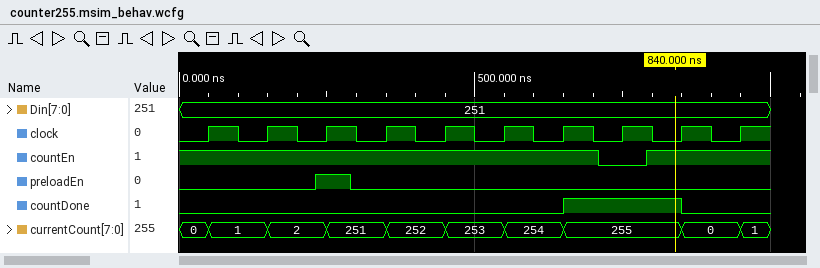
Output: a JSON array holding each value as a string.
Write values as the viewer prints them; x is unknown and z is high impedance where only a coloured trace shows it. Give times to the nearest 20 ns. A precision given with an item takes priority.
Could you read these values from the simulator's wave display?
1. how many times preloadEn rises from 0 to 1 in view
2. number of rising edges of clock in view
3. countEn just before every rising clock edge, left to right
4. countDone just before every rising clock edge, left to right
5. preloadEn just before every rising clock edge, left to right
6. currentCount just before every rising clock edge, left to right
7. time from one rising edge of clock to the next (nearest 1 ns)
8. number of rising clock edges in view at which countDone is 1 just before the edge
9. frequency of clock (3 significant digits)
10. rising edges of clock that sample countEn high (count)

["1", "10", "1 1 1 1 1 1 1 0 1 1", "0 0 0 0 0 0 0 1 1 0", "0 0 1 0 0 0 0 0 0 0", "0, 1, 2, 251, 252, 253, 254, 255, 255, 0", "100 ns", "2", "10.0 MHz", "9"]
